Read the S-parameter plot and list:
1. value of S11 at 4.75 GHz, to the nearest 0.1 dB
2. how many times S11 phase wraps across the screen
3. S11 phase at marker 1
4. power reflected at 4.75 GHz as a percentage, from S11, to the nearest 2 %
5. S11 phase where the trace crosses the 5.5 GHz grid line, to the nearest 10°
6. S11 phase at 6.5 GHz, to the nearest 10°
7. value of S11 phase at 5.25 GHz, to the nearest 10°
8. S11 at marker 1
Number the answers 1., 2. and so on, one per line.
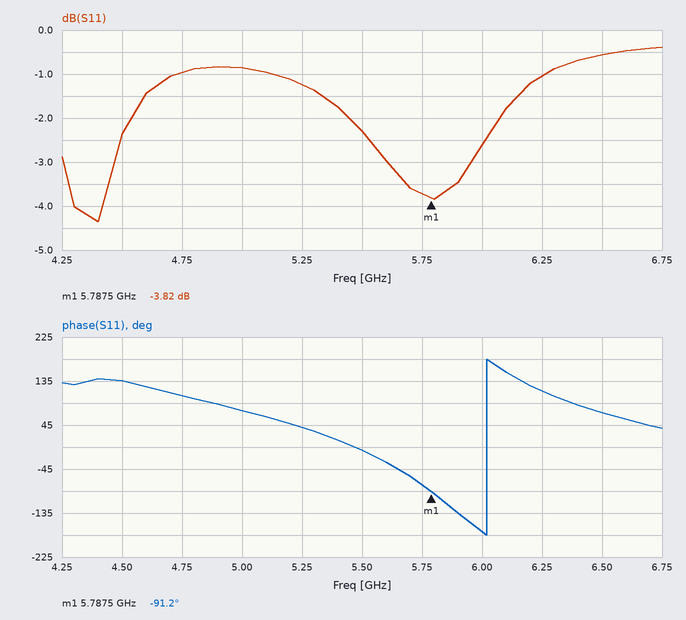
1. -1.0 dB
2. 1
3. -91.2°
4. 80 %
5. -10°
6. 70°
7. 40°
8. -3.82 dB
